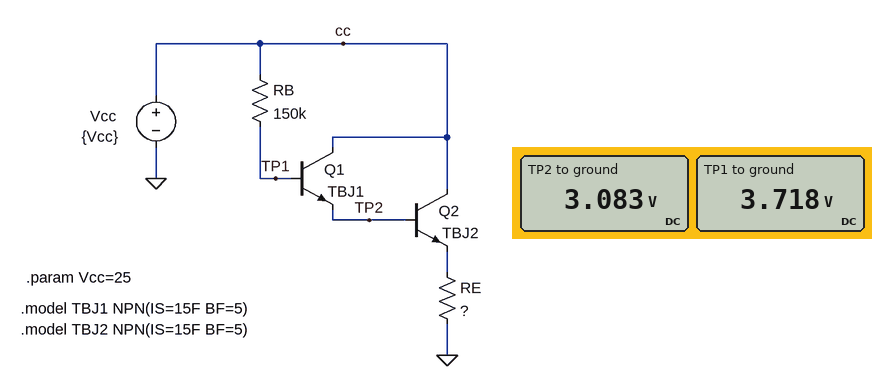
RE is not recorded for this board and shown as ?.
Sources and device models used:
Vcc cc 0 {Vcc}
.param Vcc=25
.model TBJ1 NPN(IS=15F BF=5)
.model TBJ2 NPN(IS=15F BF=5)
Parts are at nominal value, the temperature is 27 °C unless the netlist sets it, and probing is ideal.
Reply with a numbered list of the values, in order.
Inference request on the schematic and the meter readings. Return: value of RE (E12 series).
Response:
1. 470 Ω
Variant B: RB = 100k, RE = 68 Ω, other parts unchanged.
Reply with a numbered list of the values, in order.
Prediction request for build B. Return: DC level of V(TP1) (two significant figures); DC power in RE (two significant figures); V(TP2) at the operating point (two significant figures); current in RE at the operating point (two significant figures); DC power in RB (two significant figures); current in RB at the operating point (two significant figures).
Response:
1. 1.9 V
2. 4.7 mW
3. 1.3 V
4. 8.3 mA
5. 5.3 mW
6. 230 µA
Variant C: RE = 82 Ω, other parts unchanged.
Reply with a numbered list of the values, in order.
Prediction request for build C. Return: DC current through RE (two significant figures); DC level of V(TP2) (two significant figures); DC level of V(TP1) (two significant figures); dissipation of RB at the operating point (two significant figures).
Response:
1. 5.6 mA
2. 1.1 V
3. 1.8 V
4. 3.6 mW
